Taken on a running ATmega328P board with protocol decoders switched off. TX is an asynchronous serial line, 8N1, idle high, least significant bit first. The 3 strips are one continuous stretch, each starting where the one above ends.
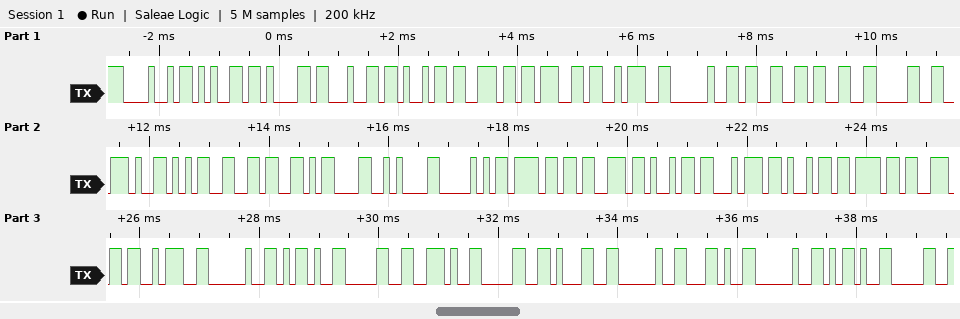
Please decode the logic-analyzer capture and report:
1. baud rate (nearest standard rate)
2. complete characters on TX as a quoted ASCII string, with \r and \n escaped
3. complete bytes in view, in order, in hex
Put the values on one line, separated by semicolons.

9600 baud; "Heading: 330.56\r\nPosition: -0.01 , -0"; 48 65 61 64 69 6E 67 3A 20 33 33 30 2E 35 36 0D 0A 50 6F 73 69 74 69 6F 6E 3A 20 2D 30 2E 30 31 20 2C 20 2D 30
